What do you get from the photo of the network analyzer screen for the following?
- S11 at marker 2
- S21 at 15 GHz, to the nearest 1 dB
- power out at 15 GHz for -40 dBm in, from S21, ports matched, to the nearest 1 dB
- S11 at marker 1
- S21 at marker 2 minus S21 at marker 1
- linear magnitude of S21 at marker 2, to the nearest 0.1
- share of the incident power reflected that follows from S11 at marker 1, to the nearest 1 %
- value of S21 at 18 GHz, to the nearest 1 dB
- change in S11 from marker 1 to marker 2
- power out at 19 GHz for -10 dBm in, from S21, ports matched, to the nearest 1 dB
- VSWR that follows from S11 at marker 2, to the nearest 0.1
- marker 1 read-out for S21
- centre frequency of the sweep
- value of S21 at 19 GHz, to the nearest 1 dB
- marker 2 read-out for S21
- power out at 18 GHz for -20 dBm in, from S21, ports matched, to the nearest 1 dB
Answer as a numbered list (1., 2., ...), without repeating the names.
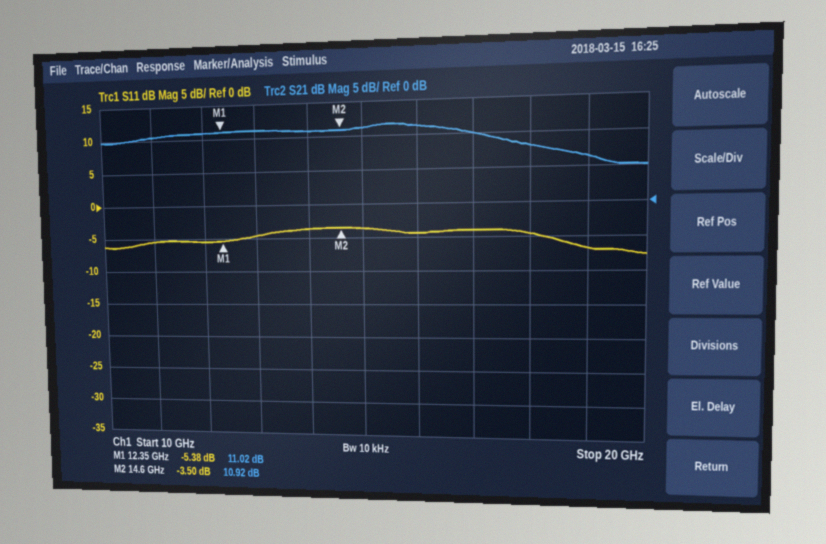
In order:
1. -3.50 dB
2. 11 dB
3. -29 dBm
4. -5.38 dB
5. -0.10 dB
6. 3.5
7. 29 %
8. 8 dB
9. 1.88 dB
10. -4 dBm
11. 5.0
12. 11.02 dB
13. 15 GHz
14. 6 dB
15. 10.92 dB
16. -12 dBm
